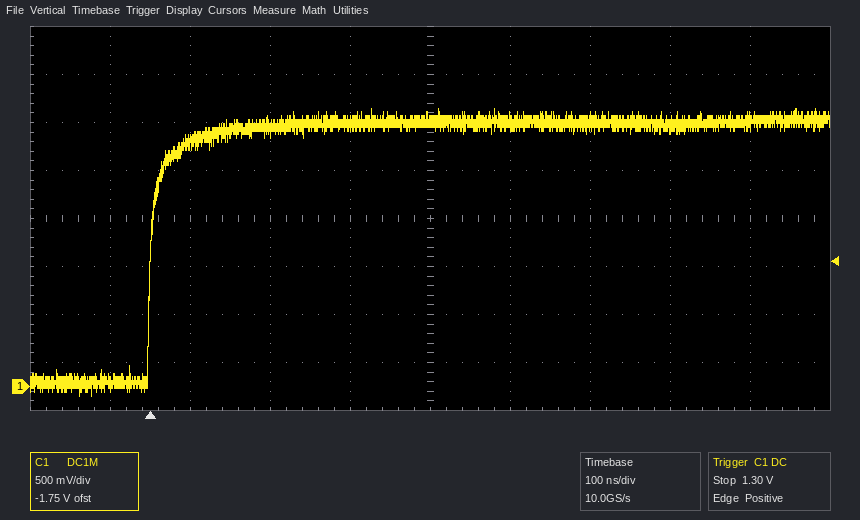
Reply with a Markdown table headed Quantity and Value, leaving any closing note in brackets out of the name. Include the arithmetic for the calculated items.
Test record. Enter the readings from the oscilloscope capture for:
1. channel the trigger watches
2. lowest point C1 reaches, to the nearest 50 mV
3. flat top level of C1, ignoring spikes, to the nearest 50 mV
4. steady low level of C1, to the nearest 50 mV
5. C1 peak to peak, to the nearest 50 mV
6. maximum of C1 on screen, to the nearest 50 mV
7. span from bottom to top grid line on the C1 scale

| Quantity | Value |
|---|---|
| channel the trigger watches | C1 |
| lowest point C1 reaches, to the nearest 50 mV | -100 mV |
| flat top level of C1, ignoring spikes, to the nearest 50 mV | 2.75 V |
| steady low level of C1, to the nearest 50 mV | 50 mV |
| C1 peak to peak, to the nearest 50 mV | 2.90 V − (-100 mV) = 3.00 V |
| maximum of C1 on screen, to the nearest 50 mV | 2.90 V |
| span from bottom to top grid line on the C1 scale | 4 V |
